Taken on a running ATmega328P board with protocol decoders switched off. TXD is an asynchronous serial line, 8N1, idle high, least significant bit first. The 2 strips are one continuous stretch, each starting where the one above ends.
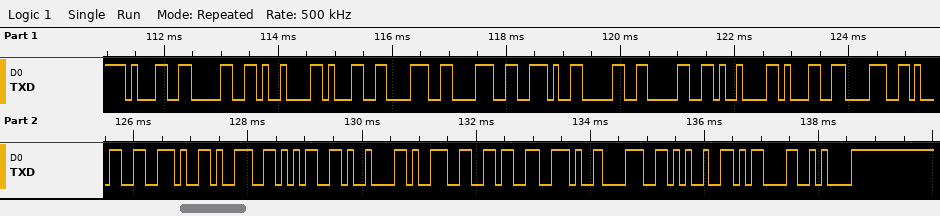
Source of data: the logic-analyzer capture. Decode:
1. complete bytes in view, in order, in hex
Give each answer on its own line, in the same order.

31 30 09 31 38 38 2E 30 30 09 31 38 31 2E 39 35 09 39 36 2E 38 25 0D 0A
